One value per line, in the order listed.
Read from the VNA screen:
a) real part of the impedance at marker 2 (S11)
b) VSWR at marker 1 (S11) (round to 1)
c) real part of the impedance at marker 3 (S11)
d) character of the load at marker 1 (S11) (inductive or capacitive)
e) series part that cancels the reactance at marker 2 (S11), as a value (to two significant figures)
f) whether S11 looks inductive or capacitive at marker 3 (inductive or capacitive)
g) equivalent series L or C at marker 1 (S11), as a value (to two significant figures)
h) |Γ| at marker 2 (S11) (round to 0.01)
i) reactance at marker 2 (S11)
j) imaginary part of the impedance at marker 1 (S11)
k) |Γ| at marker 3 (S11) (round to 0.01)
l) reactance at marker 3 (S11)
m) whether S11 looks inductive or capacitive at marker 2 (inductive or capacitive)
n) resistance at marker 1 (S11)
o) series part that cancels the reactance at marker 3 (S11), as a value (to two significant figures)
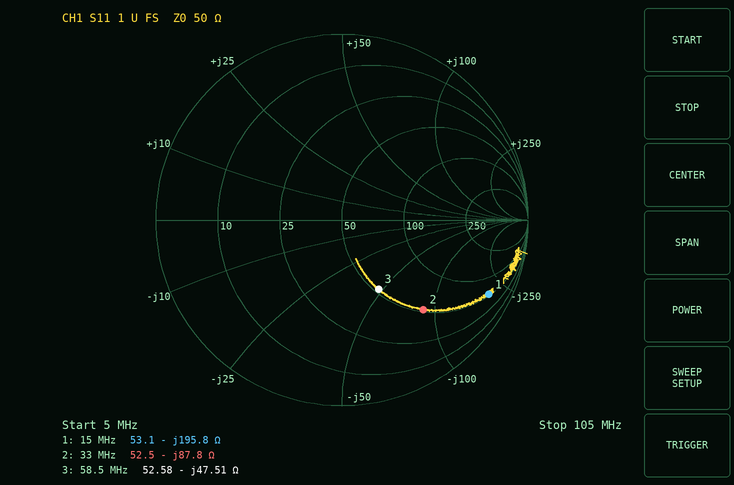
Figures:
52.5 Ω
16
52.58 Ω
capacitive
420 nH
capacitive
54 pF
0.65
-87.8 Ω
-195.8 Ω
0.42
-47.51 Ω
capacitive
53.1 Ω
130 nH
